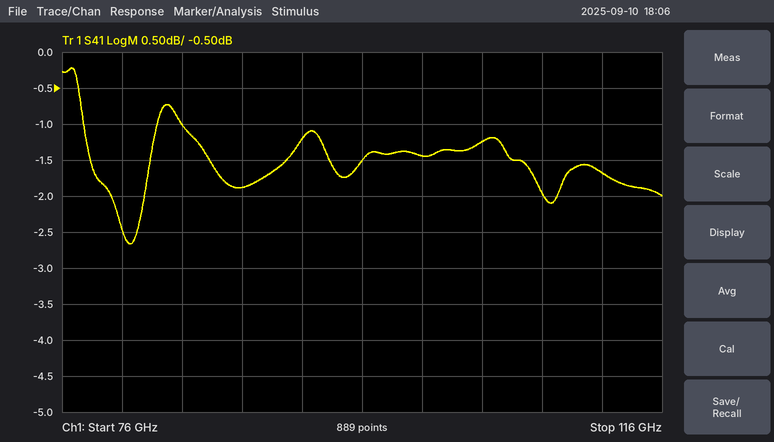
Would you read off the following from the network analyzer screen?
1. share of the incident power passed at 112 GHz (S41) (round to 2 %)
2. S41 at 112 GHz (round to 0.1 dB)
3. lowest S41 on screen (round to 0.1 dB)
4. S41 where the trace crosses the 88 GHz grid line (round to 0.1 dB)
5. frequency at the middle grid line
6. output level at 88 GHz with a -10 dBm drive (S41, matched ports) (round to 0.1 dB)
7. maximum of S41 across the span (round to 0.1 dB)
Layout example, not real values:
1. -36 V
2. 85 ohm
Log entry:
1. 68 %
2. -1.7 dB
3. -2.7 dB
4. -1.9 dB
5. 96 GHz
6. -11.9 dBm
7. -0.2 dB
